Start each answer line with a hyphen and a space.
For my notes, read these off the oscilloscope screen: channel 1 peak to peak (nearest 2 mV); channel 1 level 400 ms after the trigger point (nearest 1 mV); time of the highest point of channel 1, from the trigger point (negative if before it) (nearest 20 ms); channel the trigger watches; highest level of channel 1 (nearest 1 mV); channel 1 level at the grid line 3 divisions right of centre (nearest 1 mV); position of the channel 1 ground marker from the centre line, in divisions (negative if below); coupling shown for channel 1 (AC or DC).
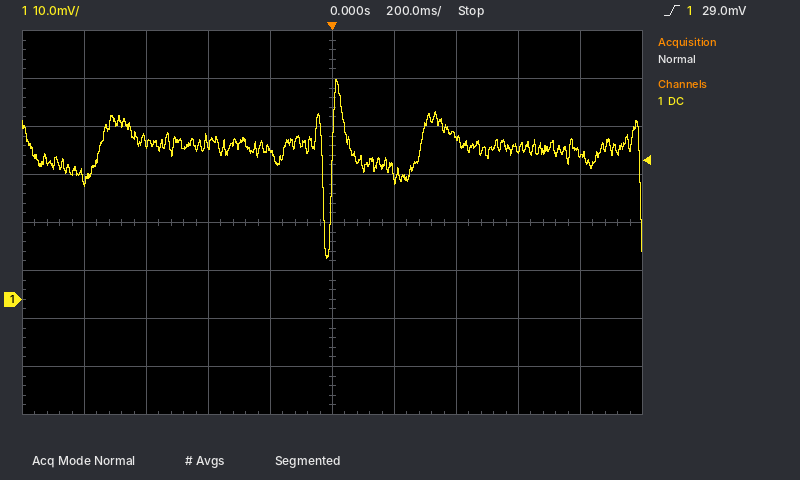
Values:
- 38 mV
- 34 mV
- +20 ms
- channel 1
- 46 mV
- 31 mV
- -1.6 div
- DC
